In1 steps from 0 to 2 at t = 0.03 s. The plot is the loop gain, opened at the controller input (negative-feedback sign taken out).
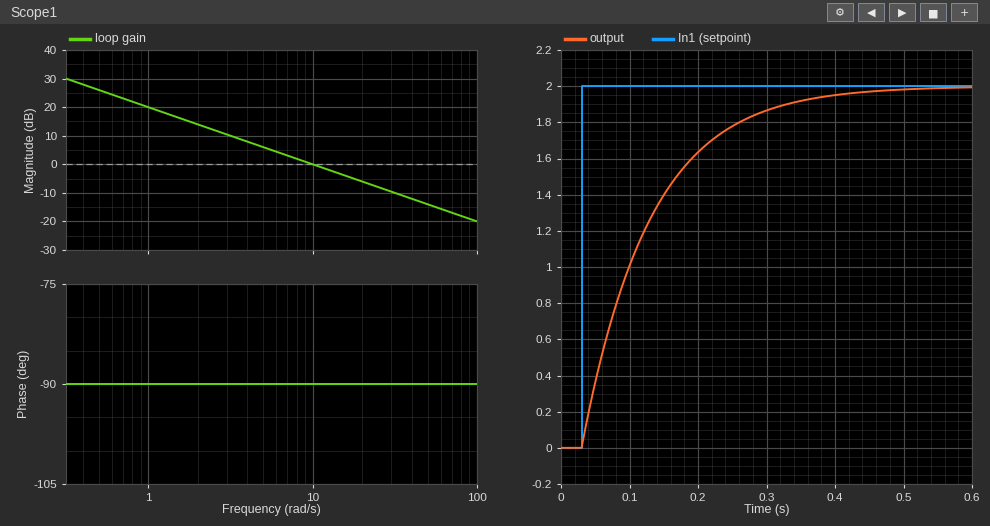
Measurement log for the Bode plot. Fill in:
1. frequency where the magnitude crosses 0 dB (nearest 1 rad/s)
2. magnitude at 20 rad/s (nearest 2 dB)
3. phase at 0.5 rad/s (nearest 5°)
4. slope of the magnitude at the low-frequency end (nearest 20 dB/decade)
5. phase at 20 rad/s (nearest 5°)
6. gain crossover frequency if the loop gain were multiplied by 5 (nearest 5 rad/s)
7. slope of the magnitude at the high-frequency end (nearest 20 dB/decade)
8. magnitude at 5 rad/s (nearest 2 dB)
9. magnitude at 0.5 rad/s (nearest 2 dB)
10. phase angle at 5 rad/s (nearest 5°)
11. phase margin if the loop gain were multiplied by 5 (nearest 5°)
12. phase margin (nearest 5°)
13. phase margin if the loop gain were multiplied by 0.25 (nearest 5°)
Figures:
10 rad/s
-6 dB
-90°
-20 dB/decade
-90°
50 rad/s
-20 dB/decade
6 dB
26 dB
-90°
90°
90°
90°
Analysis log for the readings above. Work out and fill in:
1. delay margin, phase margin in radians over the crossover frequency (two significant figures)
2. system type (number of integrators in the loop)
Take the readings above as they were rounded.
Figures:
0.16 s
1
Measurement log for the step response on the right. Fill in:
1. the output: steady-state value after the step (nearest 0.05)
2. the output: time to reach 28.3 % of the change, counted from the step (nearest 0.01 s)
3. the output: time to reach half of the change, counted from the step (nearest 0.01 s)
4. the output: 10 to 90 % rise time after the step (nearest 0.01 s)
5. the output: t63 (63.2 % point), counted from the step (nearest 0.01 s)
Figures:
2.00
0.03 s
0.07 s
0.22 s
0.10 s
